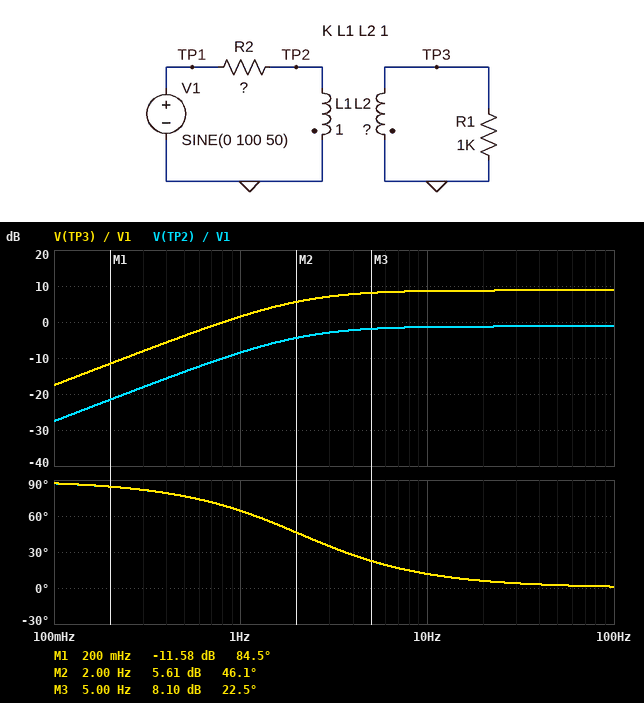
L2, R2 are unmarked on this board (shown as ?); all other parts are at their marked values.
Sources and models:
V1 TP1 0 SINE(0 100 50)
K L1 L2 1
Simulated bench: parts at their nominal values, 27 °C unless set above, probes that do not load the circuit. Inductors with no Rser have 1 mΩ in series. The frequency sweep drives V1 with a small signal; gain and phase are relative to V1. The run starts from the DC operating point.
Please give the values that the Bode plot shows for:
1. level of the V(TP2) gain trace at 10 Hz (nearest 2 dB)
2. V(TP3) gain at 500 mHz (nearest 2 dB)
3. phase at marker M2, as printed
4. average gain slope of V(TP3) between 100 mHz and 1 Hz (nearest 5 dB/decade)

-2 dB
-4 dB
46.1 deg
20 dB/decade
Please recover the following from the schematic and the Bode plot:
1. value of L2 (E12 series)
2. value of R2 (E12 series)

10 H
15 Ω
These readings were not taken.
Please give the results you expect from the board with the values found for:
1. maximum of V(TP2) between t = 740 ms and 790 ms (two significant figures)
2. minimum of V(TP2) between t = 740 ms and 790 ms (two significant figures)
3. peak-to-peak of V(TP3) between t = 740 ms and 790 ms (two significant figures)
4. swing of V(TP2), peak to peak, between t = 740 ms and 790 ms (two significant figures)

87 V
-87 V
550 V
170 V
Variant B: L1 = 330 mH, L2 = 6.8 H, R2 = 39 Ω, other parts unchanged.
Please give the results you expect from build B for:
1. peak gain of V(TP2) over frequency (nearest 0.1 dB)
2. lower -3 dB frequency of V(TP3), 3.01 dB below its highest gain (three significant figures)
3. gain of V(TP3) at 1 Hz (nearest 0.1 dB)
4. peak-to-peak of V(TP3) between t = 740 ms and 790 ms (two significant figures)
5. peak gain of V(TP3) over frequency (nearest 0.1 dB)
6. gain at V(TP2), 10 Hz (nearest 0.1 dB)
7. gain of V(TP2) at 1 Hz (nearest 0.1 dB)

-5.1 dB
10.4 Hz
-12.4 dB
490 V
8.0 dB
-8.3 dB
-25.5 dB
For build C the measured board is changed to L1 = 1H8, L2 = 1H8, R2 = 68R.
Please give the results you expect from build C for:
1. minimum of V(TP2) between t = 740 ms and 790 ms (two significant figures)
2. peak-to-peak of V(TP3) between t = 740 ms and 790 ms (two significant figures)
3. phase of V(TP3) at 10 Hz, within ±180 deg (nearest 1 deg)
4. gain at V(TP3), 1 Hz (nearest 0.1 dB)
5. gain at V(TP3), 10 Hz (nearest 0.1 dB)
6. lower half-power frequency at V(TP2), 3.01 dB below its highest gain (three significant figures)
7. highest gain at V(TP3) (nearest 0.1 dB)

-93 V
190 V
29 deg
-15.7 dB
-1.8 dB
5.63 Hz
-0.6 dB
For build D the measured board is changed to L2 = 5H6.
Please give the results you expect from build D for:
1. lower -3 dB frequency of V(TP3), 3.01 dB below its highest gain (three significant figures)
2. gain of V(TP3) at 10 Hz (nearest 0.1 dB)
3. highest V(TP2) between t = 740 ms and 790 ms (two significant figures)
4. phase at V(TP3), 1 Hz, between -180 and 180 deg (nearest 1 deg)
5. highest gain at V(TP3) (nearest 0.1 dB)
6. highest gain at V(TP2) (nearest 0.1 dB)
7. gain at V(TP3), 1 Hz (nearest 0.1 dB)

2.20 Hz
6.6 dB
92 V
66 deg
6.8 dB
-0.7 dB
-0.9 dB
